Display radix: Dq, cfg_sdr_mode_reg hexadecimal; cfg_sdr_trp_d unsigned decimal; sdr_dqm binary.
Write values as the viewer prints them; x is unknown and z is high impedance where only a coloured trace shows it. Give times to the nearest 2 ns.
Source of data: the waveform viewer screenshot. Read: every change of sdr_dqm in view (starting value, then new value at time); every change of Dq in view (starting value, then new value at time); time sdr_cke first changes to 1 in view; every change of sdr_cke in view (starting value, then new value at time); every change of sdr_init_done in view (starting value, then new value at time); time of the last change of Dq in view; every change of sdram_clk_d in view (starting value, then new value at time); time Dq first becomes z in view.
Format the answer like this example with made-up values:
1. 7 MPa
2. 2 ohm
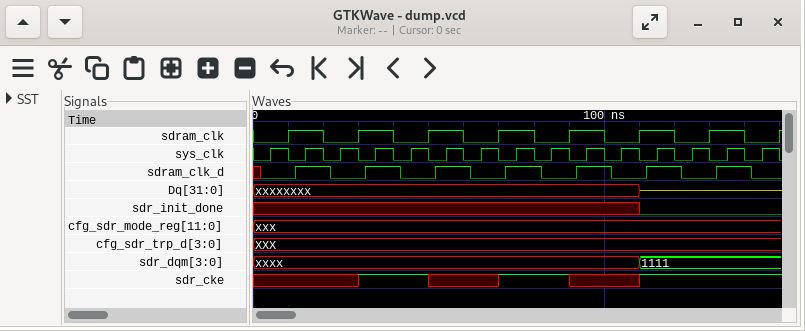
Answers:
1. xxxx, 1111 at 110 ns
2. xxxxxxxx, z at 110 ns
3. 30 ns
4. x, 1 at 30 ns, x at 50 ns, 1 at 70 ns, x at 90 ns, 1 at 110 ns
5. x, 0 at 110 ns
6. 110 ns
7. x, 0 at 2 ns, 1 at 12 ns, 0 at 22 ns, 1 at 32 ns, 0 at 42 ns, 1 at 52 ns, 0 at 62 ns, 1 at 72 ns, 0 at 82 ns, 1 at 92 ns, 0 at 102 ns, 1 at 112 ns, 0 at 122 ns, 1 at 132 ns, 0 at 142 ns
8. 110 ns
